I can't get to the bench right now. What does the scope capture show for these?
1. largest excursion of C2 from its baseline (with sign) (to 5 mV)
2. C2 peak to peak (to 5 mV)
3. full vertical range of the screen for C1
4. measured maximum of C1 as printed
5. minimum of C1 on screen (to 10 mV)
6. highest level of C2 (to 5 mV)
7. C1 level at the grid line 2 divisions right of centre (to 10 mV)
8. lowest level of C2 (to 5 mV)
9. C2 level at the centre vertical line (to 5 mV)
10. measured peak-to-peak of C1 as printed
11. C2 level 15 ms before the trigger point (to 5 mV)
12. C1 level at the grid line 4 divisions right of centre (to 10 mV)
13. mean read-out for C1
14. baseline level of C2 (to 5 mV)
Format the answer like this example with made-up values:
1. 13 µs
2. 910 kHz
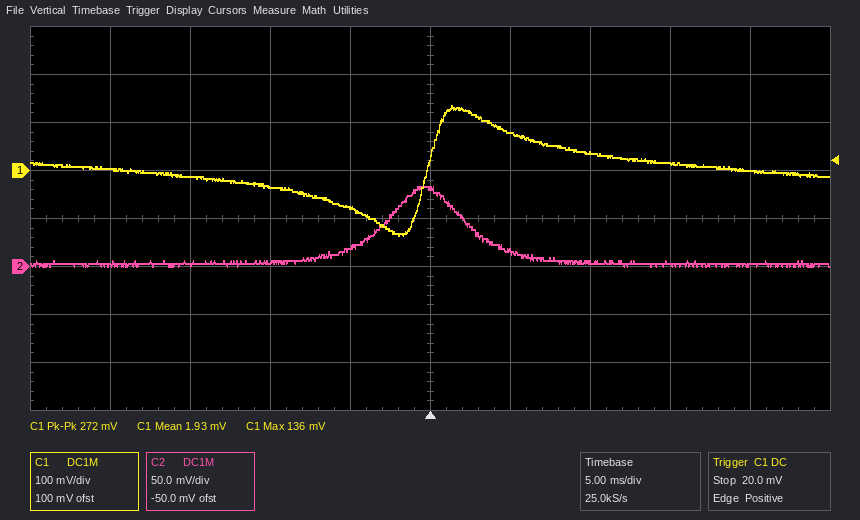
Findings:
1. +80 mV
2. 85 mV
3. 800 mV
4. 136 mV
5. -140 mV
6. 85 mV
7. 40 mV
8. 0 mV
9. 80 mV
10. 272 mV
11. 5 mV
12. 0 mV
13. 1.93 mV
14. 5 mV
